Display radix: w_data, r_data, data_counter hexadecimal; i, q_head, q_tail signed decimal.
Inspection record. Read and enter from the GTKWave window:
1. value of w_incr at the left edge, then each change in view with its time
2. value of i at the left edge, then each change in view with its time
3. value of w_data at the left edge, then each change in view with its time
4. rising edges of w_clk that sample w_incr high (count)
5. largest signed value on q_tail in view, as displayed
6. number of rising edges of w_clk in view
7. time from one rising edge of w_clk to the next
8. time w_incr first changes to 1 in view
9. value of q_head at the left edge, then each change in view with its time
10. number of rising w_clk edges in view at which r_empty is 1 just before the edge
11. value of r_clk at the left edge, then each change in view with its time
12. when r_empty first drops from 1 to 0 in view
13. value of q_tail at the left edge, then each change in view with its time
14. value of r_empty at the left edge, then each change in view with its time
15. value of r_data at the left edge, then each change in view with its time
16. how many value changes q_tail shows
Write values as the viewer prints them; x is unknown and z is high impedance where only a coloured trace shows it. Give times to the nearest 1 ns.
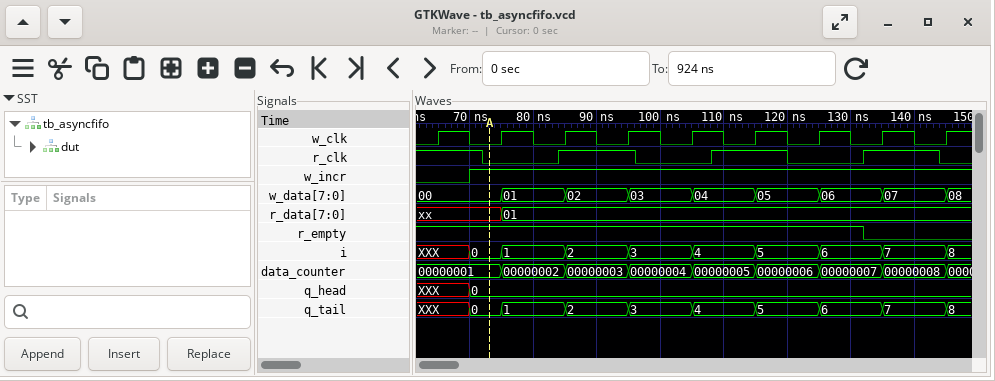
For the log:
0, 1 at 70 ns
XXX, 0 at 70 ns, 1 at 75 ns, 2 at 85 ns, 3 at 95 ns, 4 at 105 ns, 5 at 115 ns, 6 at 125 ns, 7 at 135 ns, 8 at 145 ns
00, 01 at 75 ns, 02 at 85 ns, 03 at 95 ns, 04 at 105 ns, 05 at 115 ns, 06 at 125 ns, 07 at 135 ns, 08 at 145 ns
8
8
9
10 ns
70 ns
XXX, 0 at 70 ns
7
1, 0 at 72 ns, 1 at 84 ns, 0 at 96 ns, 1 at 108 ns, 0 at 120 ns, 1 at 132 ns, 0 at 144 ns
132 ns
XXX, 0 at 70 ns, 1 at 75 ns, 2 at 85 ns, 3 at 95 ns, 4 at 105 ns, 5 at 115 ns, 6 at 125 ns, 7 at 135 ns, 8 at 145 ns
1, 0 at 132 ns
xx, 01 at 75 ns
9
